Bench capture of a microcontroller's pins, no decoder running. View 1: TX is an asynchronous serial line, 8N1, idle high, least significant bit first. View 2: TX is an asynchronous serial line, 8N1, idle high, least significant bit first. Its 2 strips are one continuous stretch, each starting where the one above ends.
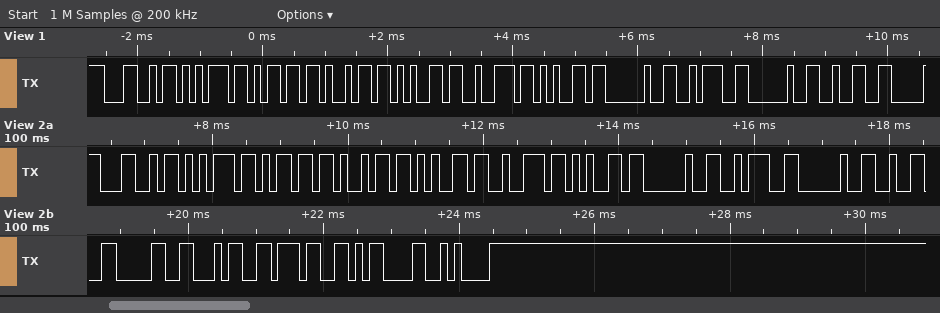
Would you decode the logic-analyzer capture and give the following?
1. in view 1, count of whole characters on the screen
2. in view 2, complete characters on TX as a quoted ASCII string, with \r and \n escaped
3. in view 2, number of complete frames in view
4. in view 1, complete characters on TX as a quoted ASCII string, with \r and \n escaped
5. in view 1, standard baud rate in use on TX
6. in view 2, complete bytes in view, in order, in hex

11
"Lumiere : 2047\r\n"
16
"Lumiere : 2"
9600 baud
4C 75 6D 69 65 72 65 20 3A 20 32 30 34 37 0D 0A
